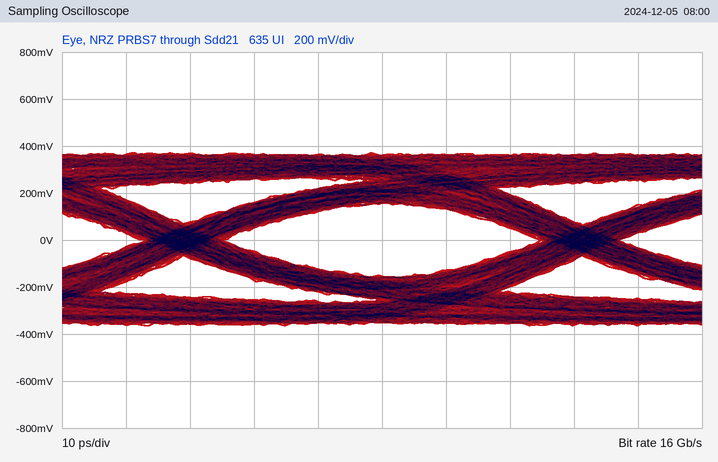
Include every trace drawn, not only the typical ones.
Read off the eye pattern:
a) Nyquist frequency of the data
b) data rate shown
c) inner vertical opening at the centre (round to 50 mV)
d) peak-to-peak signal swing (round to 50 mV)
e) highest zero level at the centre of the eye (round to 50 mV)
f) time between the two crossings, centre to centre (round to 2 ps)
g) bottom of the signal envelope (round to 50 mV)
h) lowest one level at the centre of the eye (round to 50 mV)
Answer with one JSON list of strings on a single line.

["8 GHz", "16 Gb/s", "300 mV", "750 mV", "-150 mV", "62 ps", "-350 mV", "150 mV"]
